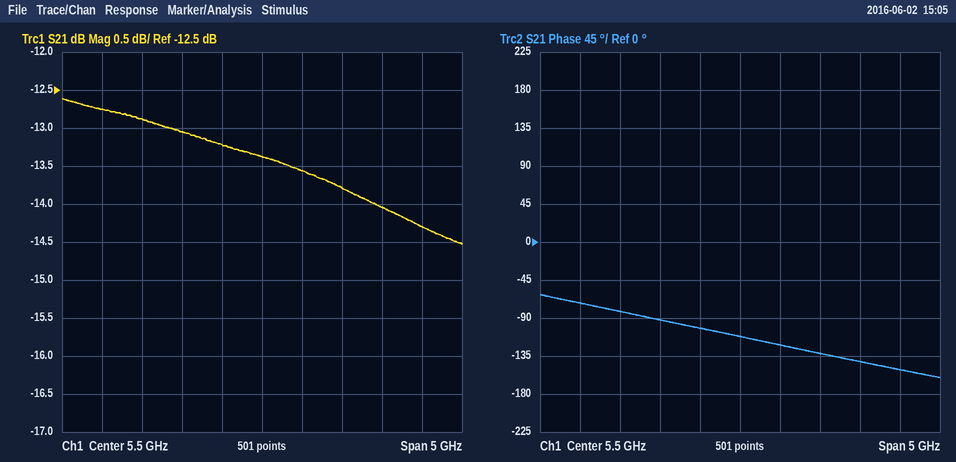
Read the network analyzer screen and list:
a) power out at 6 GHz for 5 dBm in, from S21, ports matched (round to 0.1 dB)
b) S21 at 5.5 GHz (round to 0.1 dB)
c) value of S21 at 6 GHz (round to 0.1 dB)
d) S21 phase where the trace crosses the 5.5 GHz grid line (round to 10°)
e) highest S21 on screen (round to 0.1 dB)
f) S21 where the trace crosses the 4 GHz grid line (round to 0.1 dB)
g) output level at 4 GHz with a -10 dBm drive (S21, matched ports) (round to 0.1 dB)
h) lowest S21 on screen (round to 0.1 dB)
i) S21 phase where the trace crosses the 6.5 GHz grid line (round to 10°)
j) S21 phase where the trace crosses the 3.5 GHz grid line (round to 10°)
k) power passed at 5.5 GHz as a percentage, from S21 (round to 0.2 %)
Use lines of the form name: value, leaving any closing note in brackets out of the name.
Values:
power out at 6 GHz for 5 dBm in, from S21, ports matched: -8.6 dBm
S21 at 5.5 GHz: -13.4 dB
value of S21 at 6 GHz: -13.6 dB
S21 phase where the trace crosses the 5.5 GHz grid line: -110°
highest S21 on screen: -12.6 dB
S21 where the trace crosses the 4 GHz grid line: -12.9 dB
output level at 4 GHz with a -10 dBm drive (S21, matched ports): -22.9 dBm
lowest S21 on screen: -14.5 dB
S21 phase where the trace crosses the 6.5 GHz grid line: -130°
S21 phase where the trace crosses the 3.5 GHz grid line: -70°
power passed at 5.5 GHz as a percentage, from S21: 4.6 %
